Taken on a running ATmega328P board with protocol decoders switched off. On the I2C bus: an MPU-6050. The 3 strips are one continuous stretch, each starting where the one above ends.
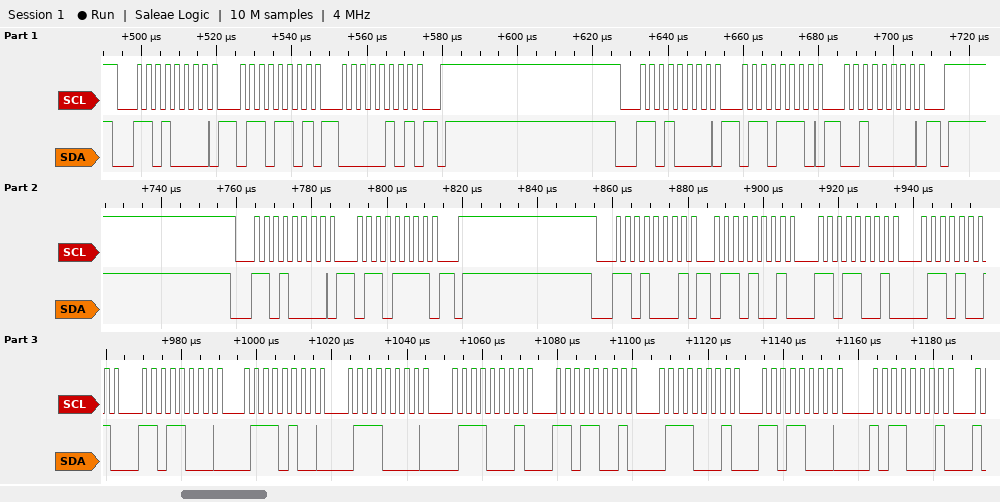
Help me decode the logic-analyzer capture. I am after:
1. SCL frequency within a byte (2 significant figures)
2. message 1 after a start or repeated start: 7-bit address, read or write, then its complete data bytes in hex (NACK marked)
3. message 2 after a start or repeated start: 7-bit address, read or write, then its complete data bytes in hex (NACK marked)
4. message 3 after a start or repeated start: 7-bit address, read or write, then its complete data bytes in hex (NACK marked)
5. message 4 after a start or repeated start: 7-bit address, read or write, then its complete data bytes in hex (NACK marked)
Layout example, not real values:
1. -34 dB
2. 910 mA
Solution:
1. 400 kHz
2. 0x68 write: 6D 05
3. 0x68 write: 6E 20
4. 0x68 write: 6F
5. 0x68 read: 69 D9 69 D8 74 70 71 D9 71 D8 B1
